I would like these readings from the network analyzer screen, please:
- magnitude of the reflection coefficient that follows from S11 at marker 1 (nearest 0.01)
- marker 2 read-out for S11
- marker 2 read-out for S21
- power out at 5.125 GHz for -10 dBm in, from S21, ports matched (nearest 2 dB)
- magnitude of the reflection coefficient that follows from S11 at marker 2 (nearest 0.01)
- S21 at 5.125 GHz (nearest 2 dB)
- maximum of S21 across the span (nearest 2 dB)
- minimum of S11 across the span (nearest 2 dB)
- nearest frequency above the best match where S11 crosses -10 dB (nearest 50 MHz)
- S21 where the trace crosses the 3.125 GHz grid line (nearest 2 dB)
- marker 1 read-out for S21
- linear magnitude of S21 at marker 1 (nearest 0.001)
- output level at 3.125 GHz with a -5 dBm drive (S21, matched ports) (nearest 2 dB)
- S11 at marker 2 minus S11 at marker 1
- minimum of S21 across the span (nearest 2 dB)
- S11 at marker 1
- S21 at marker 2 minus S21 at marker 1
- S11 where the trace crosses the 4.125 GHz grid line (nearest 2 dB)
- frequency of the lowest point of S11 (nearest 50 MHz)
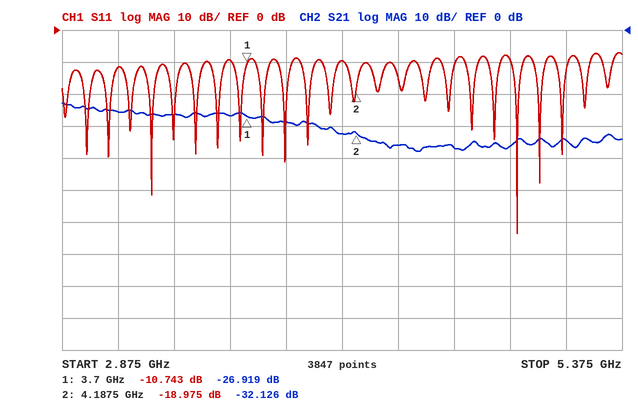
0.29
-18.975 dB
-32.126 dB
-44 dBm
0.11
-34 dB
-22 dB
-64 dB
4.95 GHz
-26 dB
-26.919 dB
0.045
-30 dBm
-8.232 dB
-38 dB
-10.743 dB
-5.207 dB
-10 dB
4.90 GHz
